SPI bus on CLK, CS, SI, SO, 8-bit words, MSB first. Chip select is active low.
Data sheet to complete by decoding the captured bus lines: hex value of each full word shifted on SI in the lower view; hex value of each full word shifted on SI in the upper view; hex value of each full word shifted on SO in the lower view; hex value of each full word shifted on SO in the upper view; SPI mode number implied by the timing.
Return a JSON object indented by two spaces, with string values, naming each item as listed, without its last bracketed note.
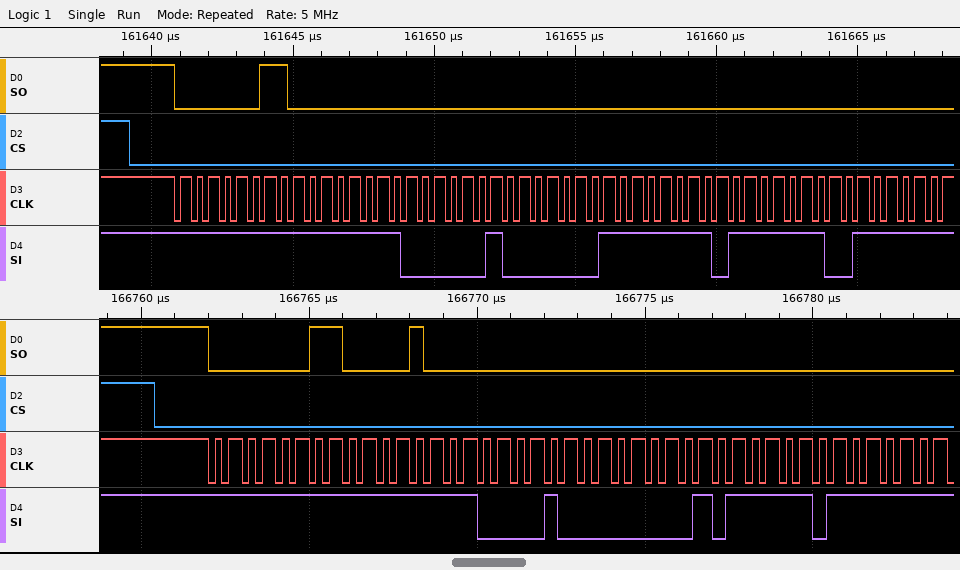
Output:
{
  "hex value of each full word shifted on SI in the lower view": "FF, FF, 08, 05, F7",
  "hex value of each full word shifted on SI in the upper view": "FF, FF, 02, 03, FD, FC",
  "hex value of each full word shifted on SO in the lower view": "03, 08, 00, 00, 00",
  "hex value of each full word shifted on SO in the upper view": "03, 00, 00, 00, 00, 00",
  "SPI mode number implied by the timing": "3"
}
